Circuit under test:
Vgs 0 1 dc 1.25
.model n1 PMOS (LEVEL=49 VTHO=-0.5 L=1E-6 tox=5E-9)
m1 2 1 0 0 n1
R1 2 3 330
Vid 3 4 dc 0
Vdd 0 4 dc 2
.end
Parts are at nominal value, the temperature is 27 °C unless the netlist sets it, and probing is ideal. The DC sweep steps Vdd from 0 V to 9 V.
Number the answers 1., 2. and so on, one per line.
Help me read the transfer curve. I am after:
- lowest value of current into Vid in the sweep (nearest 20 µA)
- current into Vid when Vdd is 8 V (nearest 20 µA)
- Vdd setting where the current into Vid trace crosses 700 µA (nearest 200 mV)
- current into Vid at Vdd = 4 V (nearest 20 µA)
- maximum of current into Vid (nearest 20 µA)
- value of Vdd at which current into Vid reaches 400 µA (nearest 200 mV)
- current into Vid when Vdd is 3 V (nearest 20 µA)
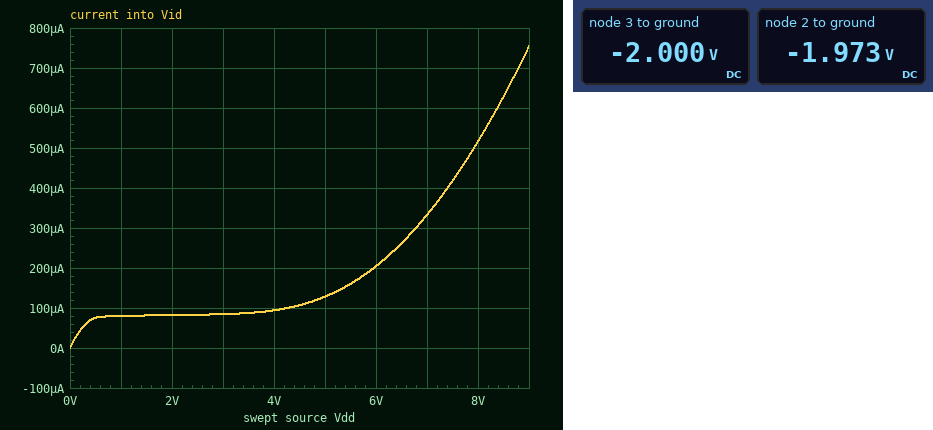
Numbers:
1. 0 A
2. 520 µA
3. 8.8 V
4. 100 µA
5. 760 µA
6. 7.4 V
7. 80 µA
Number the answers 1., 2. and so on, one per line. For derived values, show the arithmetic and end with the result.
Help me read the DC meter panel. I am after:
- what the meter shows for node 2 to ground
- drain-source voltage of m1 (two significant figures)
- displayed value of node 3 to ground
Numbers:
1. -1.973 V
2. -1.973 V = -2.0 V
3. -2.000 V
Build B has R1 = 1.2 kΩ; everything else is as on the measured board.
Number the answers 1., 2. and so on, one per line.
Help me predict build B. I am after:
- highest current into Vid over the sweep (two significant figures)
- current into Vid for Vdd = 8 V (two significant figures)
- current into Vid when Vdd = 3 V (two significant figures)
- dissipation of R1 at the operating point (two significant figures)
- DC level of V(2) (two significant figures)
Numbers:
1. 620 µA
2. 440 µA
3. 84 µA
4. 8.1 µW
5. -1.9 V
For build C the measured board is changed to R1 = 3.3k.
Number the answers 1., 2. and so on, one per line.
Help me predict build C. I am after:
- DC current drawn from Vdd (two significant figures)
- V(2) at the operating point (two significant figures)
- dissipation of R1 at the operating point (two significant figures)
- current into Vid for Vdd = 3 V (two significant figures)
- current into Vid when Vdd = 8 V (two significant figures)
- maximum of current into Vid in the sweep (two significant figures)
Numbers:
1. 82 µA
2. -1.7 V
3. 22 µW
4. 84 µA
5. 330 µA
6. 450 µA
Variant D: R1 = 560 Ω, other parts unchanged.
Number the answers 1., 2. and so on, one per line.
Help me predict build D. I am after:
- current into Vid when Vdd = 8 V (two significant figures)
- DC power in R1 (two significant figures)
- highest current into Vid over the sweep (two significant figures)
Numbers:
1. 490 µA
2. 3.8 µW
3. 710 µA
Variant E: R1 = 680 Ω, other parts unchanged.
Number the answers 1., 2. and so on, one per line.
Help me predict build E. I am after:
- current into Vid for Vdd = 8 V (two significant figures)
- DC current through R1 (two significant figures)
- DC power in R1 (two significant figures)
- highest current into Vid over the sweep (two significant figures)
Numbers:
1. 480 µA
2. 82 µA
3. 4.6 µW
4. 690 µA
